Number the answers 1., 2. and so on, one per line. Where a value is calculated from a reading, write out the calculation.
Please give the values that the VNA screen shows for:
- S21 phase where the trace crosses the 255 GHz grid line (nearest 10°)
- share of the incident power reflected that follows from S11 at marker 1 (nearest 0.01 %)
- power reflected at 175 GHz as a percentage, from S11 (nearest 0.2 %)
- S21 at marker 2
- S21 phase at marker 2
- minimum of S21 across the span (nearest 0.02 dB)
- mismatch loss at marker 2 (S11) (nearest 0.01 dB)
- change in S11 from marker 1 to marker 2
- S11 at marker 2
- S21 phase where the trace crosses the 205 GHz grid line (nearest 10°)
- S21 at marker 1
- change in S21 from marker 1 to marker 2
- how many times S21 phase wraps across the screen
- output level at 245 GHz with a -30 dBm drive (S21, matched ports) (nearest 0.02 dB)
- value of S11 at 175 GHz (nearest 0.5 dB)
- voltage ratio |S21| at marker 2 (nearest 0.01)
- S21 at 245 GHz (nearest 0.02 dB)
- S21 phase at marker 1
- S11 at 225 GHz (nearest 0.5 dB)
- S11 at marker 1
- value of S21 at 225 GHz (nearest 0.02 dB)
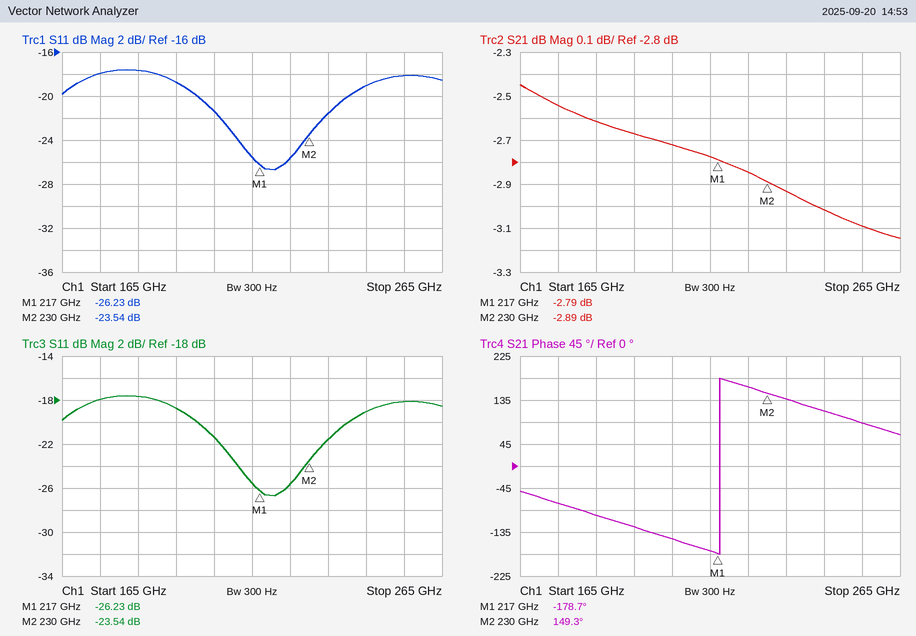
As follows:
1. 90°
2. 10^(-26.23/10) ≈ 0.24 %
3. 10^(-18/10) ≈ 1.6 %
4. -2.89 dB
5. 149.3°
6. -3.14 dB
7. −10 log10(1 − 10^(-23.54/10)) ≈ 0.02 dB
8. -23.54 − (-26.23) = 2.69 dB
9. -23.54 dB
10. -150°
11. -2.79 dB
12. -2.89 − (-2.79) = -0.10 dB
13. 1
14. -30 dBm + (-3.02 dB) = -33.02 dBm
15. -18.0 dB
16. 10^(-2.89/20) ≈ 0.72
17. -3.02 dB
18. -178.7°
19. -25.5 dB
20. -26.23 dB
21. -2.84 dB
